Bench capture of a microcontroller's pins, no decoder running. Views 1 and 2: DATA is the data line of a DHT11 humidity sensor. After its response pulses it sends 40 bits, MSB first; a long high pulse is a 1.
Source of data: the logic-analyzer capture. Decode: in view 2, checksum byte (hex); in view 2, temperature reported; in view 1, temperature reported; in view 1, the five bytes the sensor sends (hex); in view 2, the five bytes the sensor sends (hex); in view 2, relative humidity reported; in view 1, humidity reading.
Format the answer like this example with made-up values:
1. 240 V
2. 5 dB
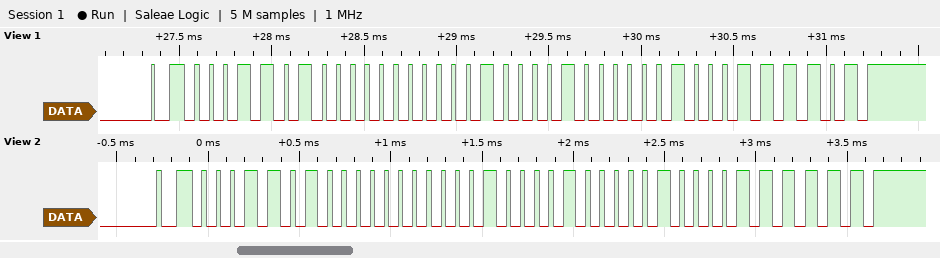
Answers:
1. 0x3F
2. 33.4 °C
3. 33.2 °C
4. 1A 00 21 02 3D
5. 1A 00 21 04 3F
6. 26 %
7. 26 %
